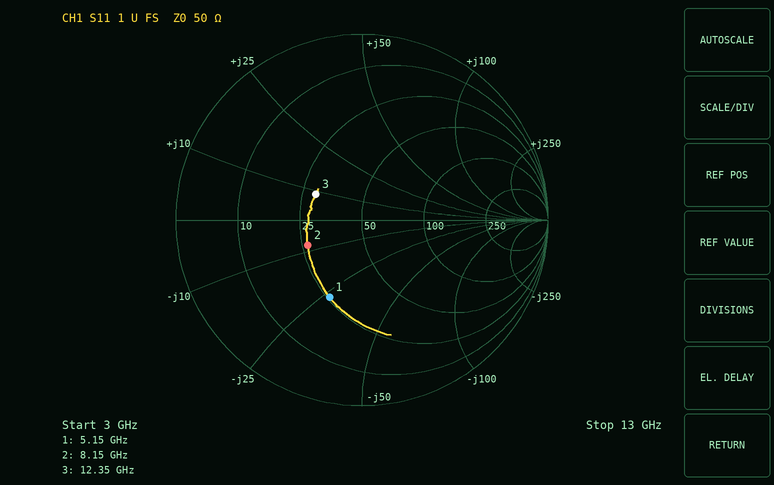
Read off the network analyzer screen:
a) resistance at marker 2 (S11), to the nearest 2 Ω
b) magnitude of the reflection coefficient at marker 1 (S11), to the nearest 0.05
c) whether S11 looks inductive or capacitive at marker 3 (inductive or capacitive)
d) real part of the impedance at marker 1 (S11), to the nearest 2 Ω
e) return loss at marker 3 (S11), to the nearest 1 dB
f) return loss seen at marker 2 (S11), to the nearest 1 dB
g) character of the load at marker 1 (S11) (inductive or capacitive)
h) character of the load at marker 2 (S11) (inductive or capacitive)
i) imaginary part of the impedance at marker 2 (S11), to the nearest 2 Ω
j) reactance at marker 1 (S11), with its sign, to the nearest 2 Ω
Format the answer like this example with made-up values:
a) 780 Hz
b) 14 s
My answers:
a) 26 Ω
b) 0.45
c) inductive
d) 26 Ω
e) 11 dB
f) 10 dB
g) capacitive
h) capacitive
i) -8 Ω
j) -26 Ω
